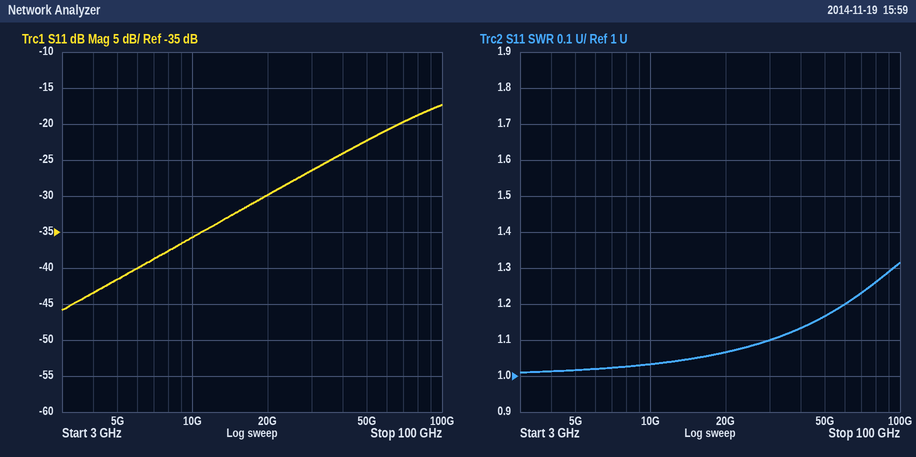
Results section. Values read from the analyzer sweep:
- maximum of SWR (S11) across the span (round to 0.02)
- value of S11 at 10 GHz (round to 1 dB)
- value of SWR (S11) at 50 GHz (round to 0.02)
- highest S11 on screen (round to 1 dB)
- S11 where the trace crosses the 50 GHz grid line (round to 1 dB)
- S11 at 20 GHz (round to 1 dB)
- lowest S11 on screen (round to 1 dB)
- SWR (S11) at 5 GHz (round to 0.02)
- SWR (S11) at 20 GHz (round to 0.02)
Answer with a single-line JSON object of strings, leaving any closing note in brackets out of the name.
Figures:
{"maximum of SWR (S11) across the span": "1.32", "value of S11 at 10 GHz": "-36 dB", "value of SWR (S11) at 50 GHz": "1.16", "highest S11 on screen": "-17 dB", "S11 where the trace crosses the 50 GHz grid line": "-22 dB", "S11 at 20 GHz": "-30 dB", "lowest S11 on screen": "-46 dB", "SWR (S11) at 5 GHz": "1.02", "SWR (S11) at 20 GHz": "1.06"}
